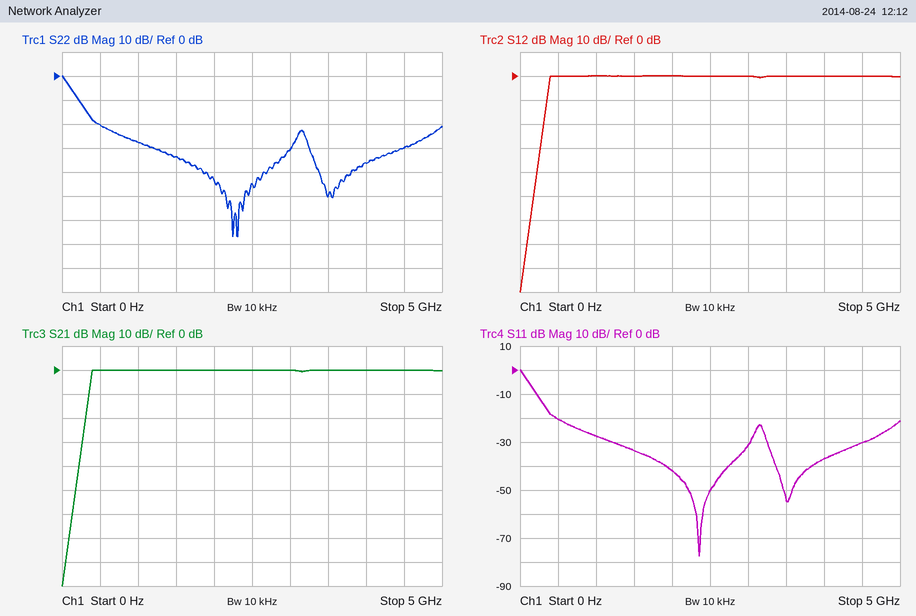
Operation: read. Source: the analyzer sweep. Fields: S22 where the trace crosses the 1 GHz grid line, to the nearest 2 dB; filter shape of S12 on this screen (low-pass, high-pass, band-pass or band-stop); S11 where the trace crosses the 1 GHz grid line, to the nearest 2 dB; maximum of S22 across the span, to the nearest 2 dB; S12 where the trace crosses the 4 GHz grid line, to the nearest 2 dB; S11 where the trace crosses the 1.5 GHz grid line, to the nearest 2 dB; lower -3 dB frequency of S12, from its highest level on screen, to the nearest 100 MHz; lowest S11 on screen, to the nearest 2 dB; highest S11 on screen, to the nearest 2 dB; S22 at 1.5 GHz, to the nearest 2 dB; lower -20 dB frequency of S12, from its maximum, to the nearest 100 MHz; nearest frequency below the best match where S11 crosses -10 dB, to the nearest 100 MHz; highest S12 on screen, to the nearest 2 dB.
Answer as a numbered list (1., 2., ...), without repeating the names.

1. -28 dB
2. high-pass
3. -28 dB
4. 0 dB
5. 0 dB
6. -34 dB
7. 400 MHz
8. -78 dB
9. 0 dB
10. -34 dB
11. 300 MHz
12. 200 MHz
13. 0 dB
